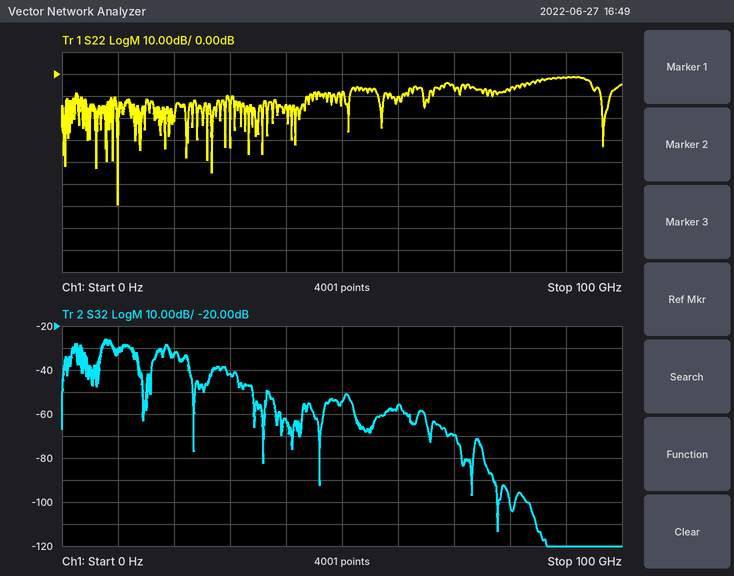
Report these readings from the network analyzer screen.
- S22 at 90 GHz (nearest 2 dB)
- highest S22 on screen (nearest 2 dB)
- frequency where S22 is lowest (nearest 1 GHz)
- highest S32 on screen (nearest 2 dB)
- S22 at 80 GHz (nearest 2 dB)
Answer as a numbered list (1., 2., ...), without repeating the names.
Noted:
1. -2 dB
2. -2 dB
3. 10 GHz
4. -26 dB
5. -8 dB
